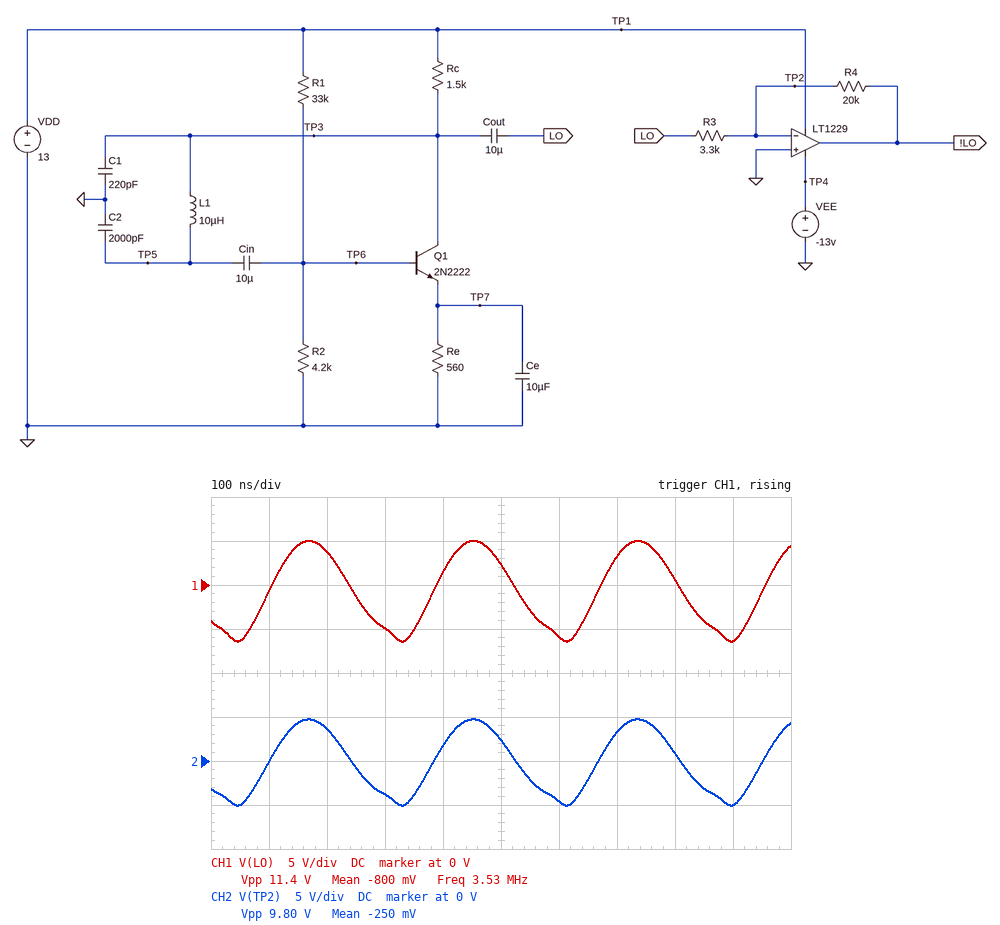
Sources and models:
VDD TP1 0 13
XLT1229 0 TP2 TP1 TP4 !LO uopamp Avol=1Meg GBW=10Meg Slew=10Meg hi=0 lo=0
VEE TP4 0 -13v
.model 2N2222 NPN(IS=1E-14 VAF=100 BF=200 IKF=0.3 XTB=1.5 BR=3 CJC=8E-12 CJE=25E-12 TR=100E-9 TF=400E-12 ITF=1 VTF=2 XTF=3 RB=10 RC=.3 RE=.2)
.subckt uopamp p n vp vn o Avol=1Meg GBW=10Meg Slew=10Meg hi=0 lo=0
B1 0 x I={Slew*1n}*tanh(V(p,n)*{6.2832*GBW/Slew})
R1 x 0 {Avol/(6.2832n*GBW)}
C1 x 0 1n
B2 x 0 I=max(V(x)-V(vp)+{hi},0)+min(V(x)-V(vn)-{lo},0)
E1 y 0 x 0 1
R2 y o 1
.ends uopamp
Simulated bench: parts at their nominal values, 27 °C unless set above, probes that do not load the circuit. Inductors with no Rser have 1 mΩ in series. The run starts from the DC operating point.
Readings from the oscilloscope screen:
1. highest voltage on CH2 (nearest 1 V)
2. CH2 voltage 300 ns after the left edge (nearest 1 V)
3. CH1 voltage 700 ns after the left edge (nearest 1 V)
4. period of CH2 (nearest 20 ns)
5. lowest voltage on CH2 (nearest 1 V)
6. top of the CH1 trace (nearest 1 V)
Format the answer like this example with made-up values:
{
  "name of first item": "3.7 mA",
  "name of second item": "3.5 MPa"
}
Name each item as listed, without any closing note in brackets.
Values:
{
  "highest voltage on CH2": "5 V",
  "CH2 voltage 300 ns after the left edge": "-4 V",
  "CH1 voltage 700 ns after the left edge": "3 V",
  "period of CH2": "280 ns",
  "lowest voltage on CH2": "-5 V",
  "top of the CH1 trace": "5 V"
}
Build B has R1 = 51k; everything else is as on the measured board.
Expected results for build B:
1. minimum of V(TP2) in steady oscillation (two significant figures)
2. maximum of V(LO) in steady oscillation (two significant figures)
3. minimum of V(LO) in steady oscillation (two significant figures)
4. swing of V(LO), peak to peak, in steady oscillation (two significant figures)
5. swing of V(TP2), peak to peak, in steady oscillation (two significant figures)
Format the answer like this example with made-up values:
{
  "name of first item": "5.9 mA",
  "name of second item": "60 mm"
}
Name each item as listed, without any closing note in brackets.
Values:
{
  "minimum of V(TP2) in steady oscillation": "-1.9 V",
  "maximum of V(LO) in steady oscillation": "2.0 V",
  "minimum of V(LO) in steady oscillation": "-2.4 V",
  "swing of V(LO), peak to peak, in steady oscillation": "4.4 V",
  "swing of V(TP2), peak to peak, in steady oscillation": "3.7 V"
}
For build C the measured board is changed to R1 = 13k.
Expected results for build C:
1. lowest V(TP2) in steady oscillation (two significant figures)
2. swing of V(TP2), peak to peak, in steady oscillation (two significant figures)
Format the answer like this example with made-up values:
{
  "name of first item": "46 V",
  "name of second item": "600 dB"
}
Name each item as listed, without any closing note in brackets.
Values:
{
  "lowest V(TP2) in steady oscillation": "-2.0 V",
  "swing of V(TP2), peak to peak, in steady oscillation": "10 V"
}
